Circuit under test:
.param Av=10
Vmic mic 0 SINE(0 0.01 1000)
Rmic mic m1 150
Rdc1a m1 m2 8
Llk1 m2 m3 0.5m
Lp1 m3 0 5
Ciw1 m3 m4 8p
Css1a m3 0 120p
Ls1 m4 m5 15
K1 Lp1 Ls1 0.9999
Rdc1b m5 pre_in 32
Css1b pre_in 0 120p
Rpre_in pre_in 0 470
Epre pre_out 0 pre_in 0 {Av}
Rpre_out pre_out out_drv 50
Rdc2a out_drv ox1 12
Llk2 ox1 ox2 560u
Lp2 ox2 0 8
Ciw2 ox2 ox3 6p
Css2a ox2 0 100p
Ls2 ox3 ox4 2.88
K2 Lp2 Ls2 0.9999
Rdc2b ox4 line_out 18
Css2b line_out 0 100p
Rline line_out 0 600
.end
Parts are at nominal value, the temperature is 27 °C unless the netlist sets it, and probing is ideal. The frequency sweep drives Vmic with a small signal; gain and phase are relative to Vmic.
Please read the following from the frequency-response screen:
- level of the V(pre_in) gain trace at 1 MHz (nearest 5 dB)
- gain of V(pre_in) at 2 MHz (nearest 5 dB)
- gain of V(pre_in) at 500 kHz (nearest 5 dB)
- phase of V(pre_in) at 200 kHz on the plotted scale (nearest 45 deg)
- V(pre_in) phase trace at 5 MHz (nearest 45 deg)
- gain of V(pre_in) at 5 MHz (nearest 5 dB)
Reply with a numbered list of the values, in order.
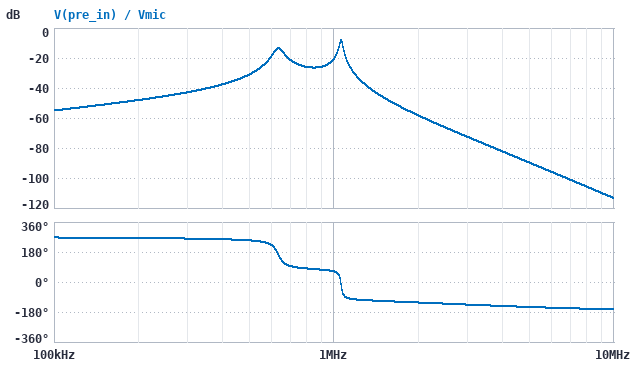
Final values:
1. -20 dB
2. -60 dB
3. -30 dB
4. 270 deg
5. -135 deg
6. -90 dB
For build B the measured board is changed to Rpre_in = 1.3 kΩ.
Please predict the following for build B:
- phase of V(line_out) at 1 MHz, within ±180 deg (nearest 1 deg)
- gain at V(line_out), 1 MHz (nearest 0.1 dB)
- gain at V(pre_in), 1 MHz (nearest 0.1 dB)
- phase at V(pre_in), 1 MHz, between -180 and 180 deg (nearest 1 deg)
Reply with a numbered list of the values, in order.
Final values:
1. -74 deg
2. -37.8 dB
3. -15.7 dB
4. 36 deg
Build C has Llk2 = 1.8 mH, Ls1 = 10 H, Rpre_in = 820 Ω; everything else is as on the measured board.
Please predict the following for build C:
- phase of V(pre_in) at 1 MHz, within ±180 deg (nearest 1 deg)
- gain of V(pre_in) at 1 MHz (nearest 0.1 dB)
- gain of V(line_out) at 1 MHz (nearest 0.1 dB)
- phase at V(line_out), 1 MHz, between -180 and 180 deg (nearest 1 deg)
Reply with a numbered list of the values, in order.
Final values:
1. 59 deg
2. -31.7 dB
3. -67.8 dB
4. -53 deg
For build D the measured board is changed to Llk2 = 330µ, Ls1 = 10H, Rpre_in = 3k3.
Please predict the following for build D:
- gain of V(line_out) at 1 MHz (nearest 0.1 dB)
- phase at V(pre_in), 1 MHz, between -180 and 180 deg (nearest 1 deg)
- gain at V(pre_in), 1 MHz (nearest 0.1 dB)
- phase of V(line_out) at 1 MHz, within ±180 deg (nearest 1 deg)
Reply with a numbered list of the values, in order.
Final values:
1. -37.9 dB
2. 24 deg
3. -27.6 dB
4. -81 deg
